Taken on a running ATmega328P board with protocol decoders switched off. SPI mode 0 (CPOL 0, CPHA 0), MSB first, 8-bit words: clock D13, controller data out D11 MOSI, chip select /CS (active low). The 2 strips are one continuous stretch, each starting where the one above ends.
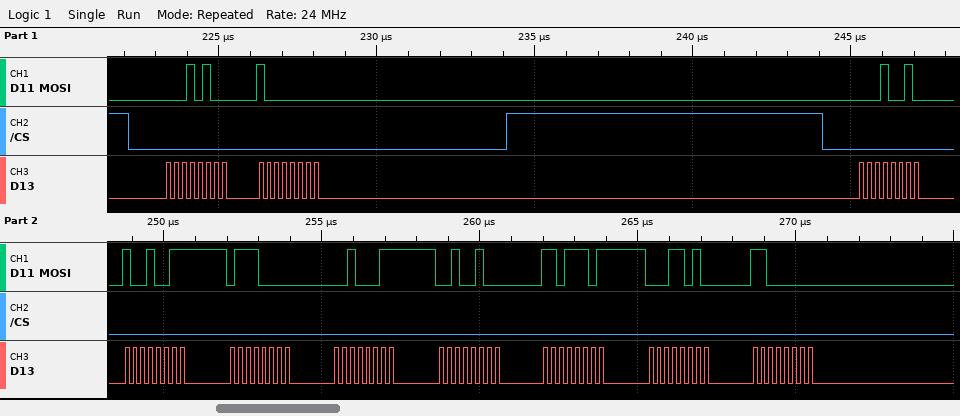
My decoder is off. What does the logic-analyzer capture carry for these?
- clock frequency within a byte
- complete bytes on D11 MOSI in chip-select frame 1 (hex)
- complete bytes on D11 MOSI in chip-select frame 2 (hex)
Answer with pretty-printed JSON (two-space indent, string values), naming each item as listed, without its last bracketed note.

{
  "clock frequency within a byte": "4 MHz",
  "complete bytes on D11 MOSI in chip-select frame 1": "0x14 0x80",
  "complete bytes on D11 MOSI in chip-select frame 2": "0x12 0x93 0x70 0x23 0x24 0xDD 0x1A 0xC0"
}
